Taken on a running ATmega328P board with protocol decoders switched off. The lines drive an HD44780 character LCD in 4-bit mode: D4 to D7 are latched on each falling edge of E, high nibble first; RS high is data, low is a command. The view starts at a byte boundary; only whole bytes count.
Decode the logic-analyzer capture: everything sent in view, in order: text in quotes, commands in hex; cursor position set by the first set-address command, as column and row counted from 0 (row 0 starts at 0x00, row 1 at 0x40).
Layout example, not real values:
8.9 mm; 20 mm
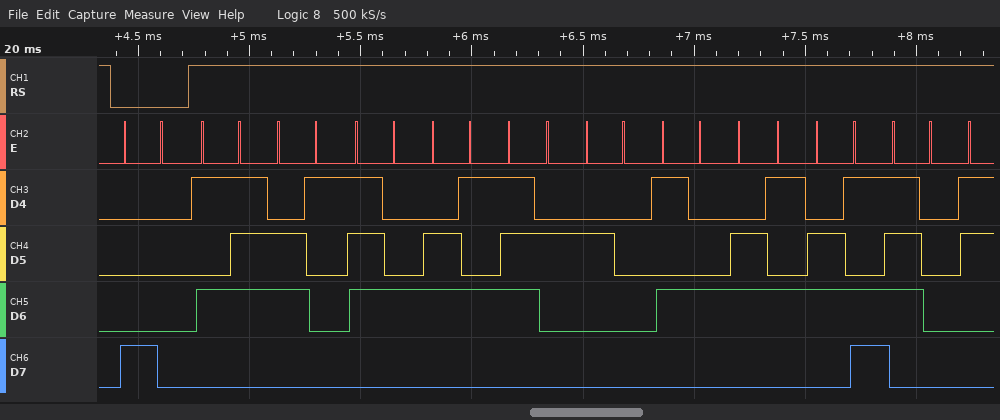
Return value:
0x80 "Water Temp"; column 0, row 0
